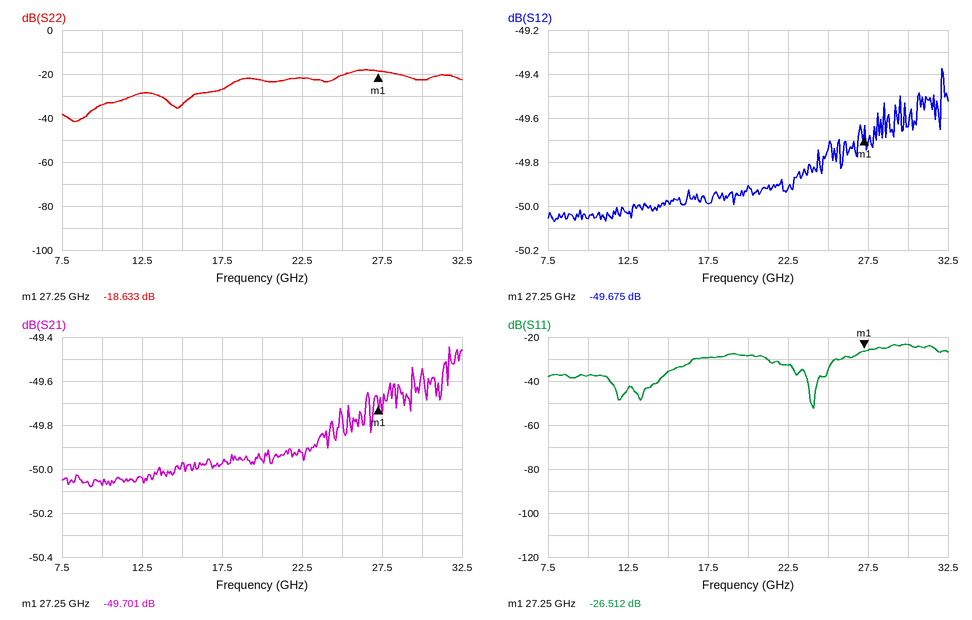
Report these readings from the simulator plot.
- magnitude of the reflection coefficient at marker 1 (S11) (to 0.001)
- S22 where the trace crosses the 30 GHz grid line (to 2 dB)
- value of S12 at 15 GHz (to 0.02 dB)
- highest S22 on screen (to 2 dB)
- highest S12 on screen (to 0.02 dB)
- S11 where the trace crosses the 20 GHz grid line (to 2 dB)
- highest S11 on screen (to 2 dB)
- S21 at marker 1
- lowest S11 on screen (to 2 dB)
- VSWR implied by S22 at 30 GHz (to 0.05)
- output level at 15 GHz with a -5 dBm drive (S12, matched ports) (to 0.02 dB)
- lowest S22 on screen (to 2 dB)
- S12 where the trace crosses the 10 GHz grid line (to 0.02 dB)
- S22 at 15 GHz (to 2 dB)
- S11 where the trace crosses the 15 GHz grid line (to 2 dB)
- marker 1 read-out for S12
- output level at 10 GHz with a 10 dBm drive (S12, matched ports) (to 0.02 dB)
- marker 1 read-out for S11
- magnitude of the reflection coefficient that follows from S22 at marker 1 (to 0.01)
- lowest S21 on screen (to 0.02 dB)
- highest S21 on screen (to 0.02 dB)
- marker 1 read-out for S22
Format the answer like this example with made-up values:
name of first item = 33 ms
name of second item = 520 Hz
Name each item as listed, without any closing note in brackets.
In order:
magnitude of the reflection coefficient at marker 1 (S11) = 0.047
S22 where the trace crosses the 30 GHz grid line = -22 dB
value of S12 at 15 GHz = -49.98 dB
highest S22 on screen = -18 dB
highest S12 on screen = -49.38 dB
S11 where the trace crosses the 20 GHz grid line = -28 dB
highest S11 on screen = -24 dB
S21 at marker 1 = -49.701 dB
lowest S11 on screen = -52 dB
VSWR implied by S22 at 30 GHz = 1.15
output level at 15 GHz with a -5 dBm drive (S12, matched ports) = -54.98 dBm
lowest S22 on screen = -42 dB
S12 where the trace crosses the 10 GHz grid line = -50.06 dB
S22 at 15 GHz = -34 dB
S11 where the trace crosses the 15 GHz grid line = -36 dB
marker 1 read-out for S12 = -49.675 dB
output level at 10 GHz with a 10 dBm drive (S12, matched ports) = -40.06 dBm
marker 1 read-out for S11 = -26.512 dB
magnitude of the reflection coefficient that follows from S22 at marker 1 = 0.12
lowest S21 on screen = -50.08 dB
highest S21 on screen = -49.44 dB
marker 1 read-out for S22 = -18.633 dB
